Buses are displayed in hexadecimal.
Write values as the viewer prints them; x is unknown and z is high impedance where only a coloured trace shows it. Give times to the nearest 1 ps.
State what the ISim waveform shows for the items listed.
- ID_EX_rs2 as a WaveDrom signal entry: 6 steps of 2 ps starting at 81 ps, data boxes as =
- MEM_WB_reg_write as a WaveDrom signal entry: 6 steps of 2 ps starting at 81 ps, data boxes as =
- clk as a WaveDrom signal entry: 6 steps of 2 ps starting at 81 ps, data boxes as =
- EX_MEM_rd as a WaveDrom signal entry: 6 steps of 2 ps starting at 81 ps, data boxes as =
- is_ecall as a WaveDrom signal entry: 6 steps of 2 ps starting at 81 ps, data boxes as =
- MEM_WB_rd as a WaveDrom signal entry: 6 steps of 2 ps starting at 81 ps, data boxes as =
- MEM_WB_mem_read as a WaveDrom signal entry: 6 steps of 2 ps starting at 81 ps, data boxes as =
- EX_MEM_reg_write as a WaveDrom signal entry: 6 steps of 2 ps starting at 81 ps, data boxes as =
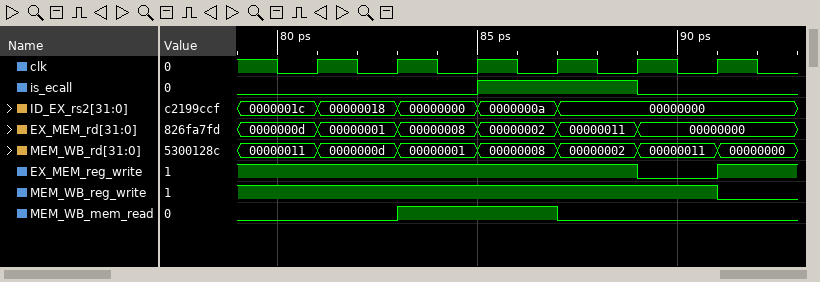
{name: 'ID_EX_rs2', wave: '====..', data: '00000018 00000000 0000000a 00000000'}
{name: 'MEM_WB_reg_write', wave: '1....0'}
{name: 'clk', wave: 'p.....'}
{name: 'EX_MEM_rd', wave: '=====.', data: '00000001 00000008 00000002 00000011 00000000'}
{name: 'is_ecall', wave: '0.1.0.'}
{name: 'MEM_WB_rd', wave: '======', data: '0000000d 00000001 00000008 00000002 00000011 00000000'}
{name: 'MEM_WB_mem_read', wave: '01.0..'}
{name: 'EX_MEM_reg_write', wave: '1...01'}
